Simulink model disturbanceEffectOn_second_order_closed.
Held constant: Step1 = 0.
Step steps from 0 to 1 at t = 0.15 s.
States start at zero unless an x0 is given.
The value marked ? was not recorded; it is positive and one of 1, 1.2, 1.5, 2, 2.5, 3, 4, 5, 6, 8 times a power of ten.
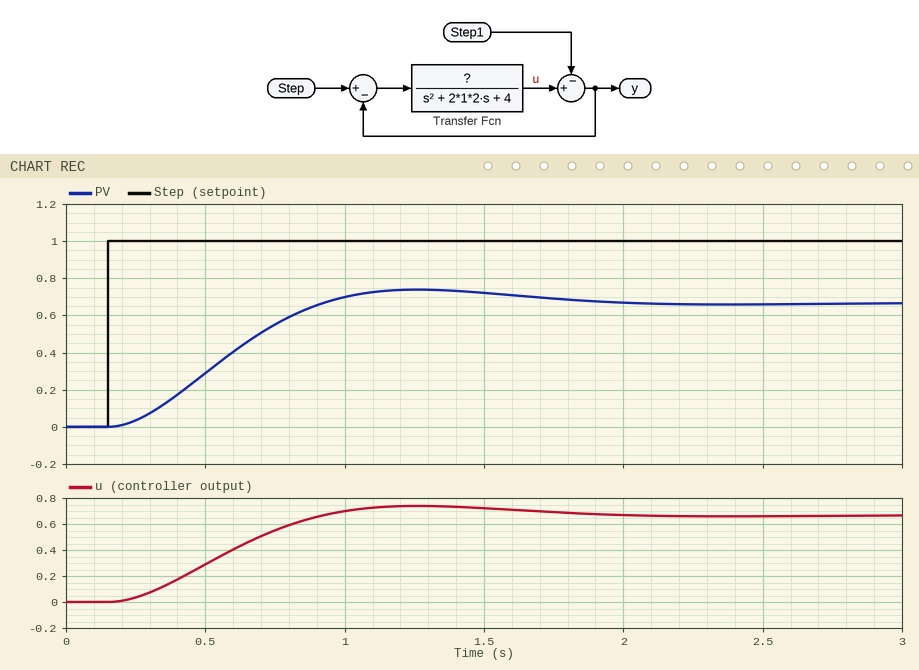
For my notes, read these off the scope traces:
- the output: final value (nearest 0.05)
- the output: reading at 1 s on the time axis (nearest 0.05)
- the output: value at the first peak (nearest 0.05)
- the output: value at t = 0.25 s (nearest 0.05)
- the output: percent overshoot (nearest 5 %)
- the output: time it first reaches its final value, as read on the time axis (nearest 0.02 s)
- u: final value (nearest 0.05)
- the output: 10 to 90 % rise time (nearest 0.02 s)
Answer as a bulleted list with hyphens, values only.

- 0.65
- 0.70
- 0.75
- 0.05
- 10 %
- 0.92 s
- 0.65
- 0.52 s
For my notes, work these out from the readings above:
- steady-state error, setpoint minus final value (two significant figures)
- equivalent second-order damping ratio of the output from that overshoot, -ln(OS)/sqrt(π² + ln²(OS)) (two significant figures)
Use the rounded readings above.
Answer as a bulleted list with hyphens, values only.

- 0.35
- 0.59
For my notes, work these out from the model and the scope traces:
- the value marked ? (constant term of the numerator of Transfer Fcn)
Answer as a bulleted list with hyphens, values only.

- 8
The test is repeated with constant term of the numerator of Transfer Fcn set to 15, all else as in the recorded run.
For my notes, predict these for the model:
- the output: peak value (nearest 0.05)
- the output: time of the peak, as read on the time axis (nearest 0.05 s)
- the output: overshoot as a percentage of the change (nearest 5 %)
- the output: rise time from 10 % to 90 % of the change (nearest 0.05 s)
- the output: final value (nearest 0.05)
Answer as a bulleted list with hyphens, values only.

- 0.95
- 0.95 s
- 20 %
- 0.35 s
- 0.80
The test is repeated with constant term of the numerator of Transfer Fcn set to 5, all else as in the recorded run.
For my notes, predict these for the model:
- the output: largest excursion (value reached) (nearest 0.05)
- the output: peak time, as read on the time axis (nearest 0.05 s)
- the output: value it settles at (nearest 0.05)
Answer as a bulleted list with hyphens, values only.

- 0.60
- 1.55 s
- 0.55
